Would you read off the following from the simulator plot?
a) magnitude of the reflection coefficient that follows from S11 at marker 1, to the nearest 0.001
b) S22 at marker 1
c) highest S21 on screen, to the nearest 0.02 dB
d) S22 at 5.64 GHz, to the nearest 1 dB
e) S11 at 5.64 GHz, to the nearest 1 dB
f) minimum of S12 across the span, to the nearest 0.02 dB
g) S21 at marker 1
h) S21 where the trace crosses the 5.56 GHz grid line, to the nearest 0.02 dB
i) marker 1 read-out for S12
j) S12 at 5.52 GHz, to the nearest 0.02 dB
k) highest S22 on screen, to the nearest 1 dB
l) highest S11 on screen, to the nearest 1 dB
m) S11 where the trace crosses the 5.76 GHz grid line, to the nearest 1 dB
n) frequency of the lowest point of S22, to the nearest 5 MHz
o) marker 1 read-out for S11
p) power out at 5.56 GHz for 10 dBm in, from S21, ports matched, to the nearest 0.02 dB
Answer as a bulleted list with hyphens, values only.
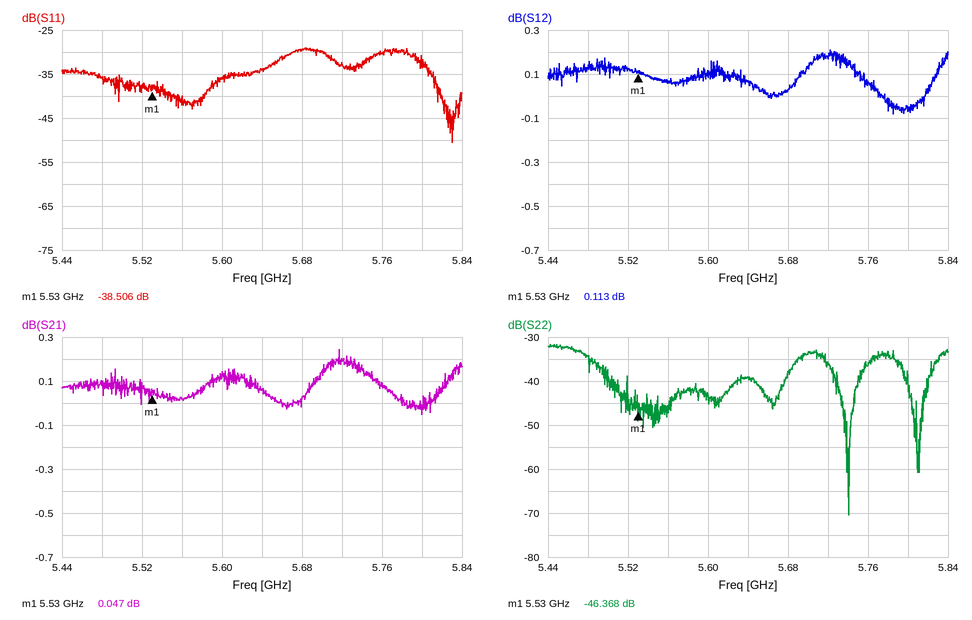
- 0.012
- -46.368 dB
- 0.24 dB
- -39 dB
- -34 dB
- -0.08 dB
- 0.047 dB
- 0.02 dB
- 0.113 dB
- 0.12 dB
- -32 dB
- -29 dB
- -30 dB
- 5.740 GHz
- -38.506 dB
- 10.02 dBm
